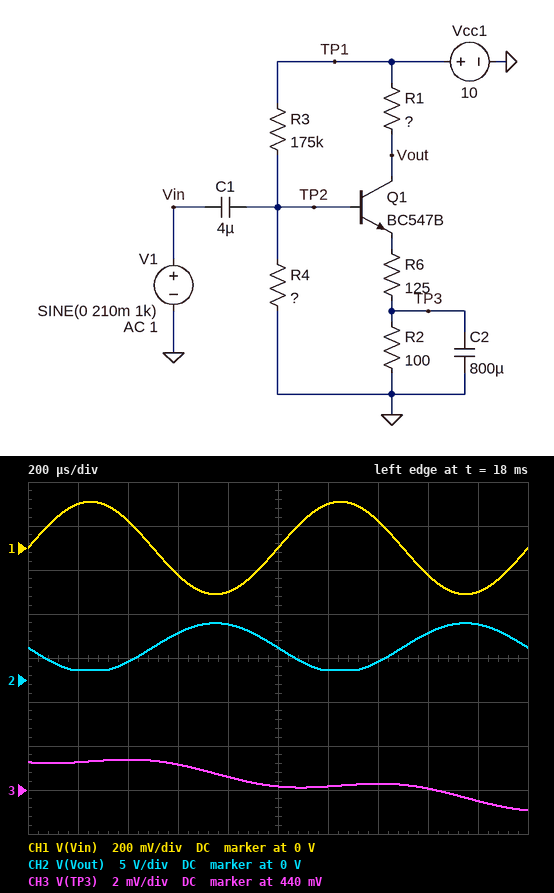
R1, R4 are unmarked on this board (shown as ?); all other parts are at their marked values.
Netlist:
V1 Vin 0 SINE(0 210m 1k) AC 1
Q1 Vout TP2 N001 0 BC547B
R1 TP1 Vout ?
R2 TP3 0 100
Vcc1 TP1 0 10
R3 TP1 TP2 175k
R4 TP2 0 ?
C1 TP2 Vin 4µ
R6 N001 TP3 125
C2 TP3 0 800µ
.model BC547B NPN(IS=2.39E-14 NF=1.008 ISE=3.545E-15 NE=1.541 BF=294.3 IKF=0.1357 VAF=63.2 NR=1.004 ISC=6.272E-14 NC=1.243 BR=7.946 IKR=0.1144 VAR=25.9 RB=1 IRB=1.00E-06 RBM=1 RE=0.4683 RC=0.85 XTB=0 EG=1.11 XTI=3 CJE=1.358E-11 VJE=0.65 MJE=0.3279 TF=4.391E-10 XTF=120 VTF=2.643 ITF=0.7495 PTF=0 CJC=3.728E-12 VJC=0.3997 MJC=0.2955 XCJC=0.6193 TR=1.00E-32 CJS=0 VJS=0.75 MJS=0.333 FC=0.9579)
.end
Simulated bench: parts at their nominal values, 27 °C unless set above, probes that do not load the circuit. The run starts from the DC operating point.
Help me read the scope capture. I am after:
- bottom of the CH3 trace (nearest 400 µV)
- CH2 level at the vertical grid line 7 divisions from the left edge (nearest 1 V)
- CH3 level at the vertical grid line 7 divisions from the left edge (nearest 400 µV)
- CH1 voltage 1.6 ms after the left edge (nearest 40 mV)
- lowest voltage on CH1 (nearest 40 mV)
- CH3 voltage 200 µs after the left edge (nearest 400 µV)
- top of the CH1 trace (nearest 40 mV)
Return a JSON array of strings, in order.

["439.2 mV", "2 V", "440.4 mV", "-120 mV", "-200 mV", "441.2 mV", "200 mV"]
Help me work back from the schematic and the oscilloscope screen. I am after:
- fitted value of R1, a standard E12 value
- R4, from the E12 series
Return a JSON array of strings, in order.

["1.8 kΩ", "56 kΩ"]
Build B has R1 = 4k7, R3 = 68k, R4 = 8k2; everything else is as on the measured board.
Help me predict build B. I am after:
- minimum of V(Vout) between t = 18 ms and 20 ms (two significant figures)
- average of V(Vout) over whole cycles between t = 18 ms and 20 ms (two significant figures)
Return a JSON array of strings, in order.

["470 mV", "5.5 V"]
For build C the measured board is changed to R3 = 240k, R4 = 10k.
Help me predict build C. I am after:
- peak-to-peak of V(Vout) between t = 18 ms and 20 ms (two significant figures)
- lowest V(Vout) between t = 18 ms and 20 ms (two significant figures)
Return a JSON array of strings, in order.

["300 mV", "9.7 V"]
